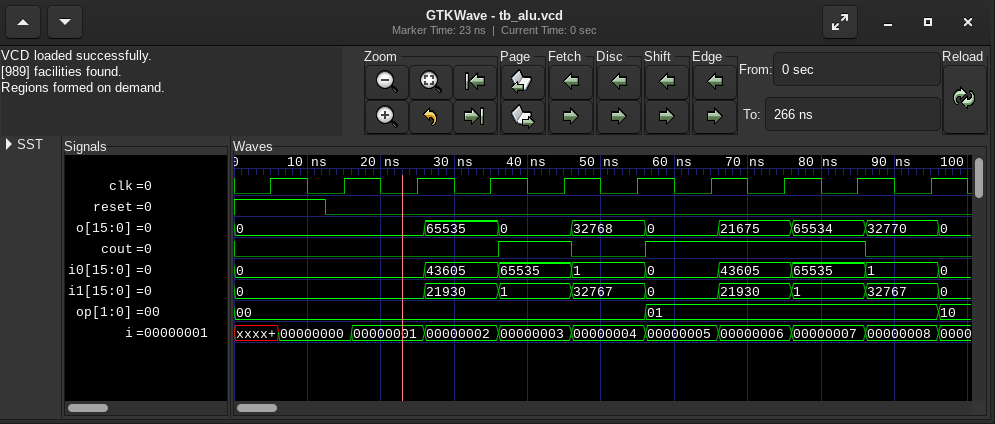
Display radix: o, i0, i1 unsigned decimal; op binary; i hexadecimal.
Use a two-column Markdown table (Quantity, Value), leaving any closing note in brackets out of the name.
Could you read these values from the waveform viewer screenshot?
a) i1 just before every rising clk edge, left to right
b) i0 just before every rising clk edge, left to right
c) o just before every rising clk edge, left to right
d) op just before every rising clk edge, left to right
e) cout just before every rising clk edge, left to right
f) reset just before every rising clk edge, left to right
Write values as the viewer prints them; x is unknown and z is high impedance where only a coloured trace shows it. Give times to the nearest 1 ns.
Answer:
| Quantity | Value |
|---|---|
| i1 just before every rising clk edge, left to right | 0, 0, 0, 21930, 1, 32767, 0, 21930, 1, 32767 |
| i0 just before every rising clk edge, left to right | 0, 0, 0, 43605, 65535, 1, 0, 43605, 65535, 1 |
| o just before every rising clk edge, left to right | 0, 0, 0, 65535, 0, 32768, 0, 21675, 65534, 32770 |
| op just before every rising clk edge, left to right | 00, 00, 00, 00, 00, 00, 01, 01, 01, 01 |
| cout just before every rising clk edge, left to right | 0 0 0 0 1 0 1 1 1 0 |
| reset just before every rising clk edge, left to right | 1 0 0 0 0 0 0 0 0 0 |
